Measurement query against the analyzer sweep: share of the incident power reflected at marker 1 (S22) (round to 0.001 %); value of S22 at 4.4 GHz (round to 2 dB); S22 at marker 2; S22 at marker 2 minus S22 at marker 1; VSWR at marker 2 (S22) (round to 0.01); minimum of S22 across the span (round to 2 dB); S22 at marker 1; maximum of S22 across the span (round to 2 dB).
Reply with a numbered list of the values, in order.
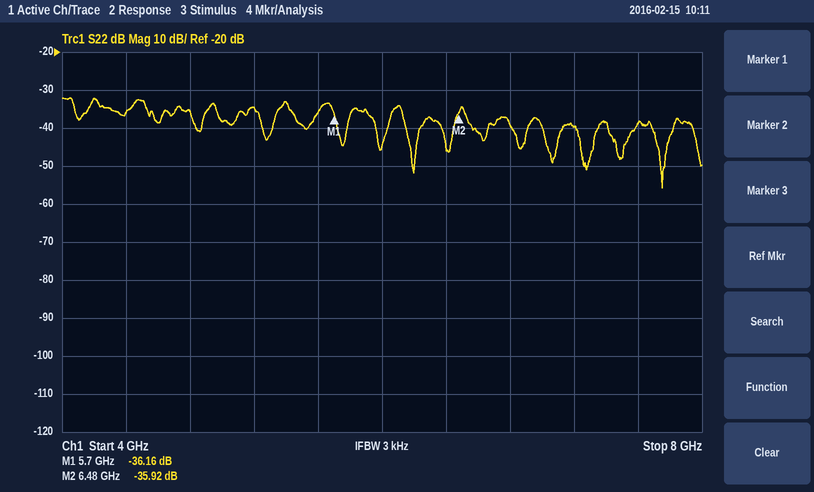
1. 0.024 %
2. -36 dB
3. -35.92 dB
4. 0.24 dB
5. 1.03
6. -56 dB
7. -36.16 dB
8. -32 dB
